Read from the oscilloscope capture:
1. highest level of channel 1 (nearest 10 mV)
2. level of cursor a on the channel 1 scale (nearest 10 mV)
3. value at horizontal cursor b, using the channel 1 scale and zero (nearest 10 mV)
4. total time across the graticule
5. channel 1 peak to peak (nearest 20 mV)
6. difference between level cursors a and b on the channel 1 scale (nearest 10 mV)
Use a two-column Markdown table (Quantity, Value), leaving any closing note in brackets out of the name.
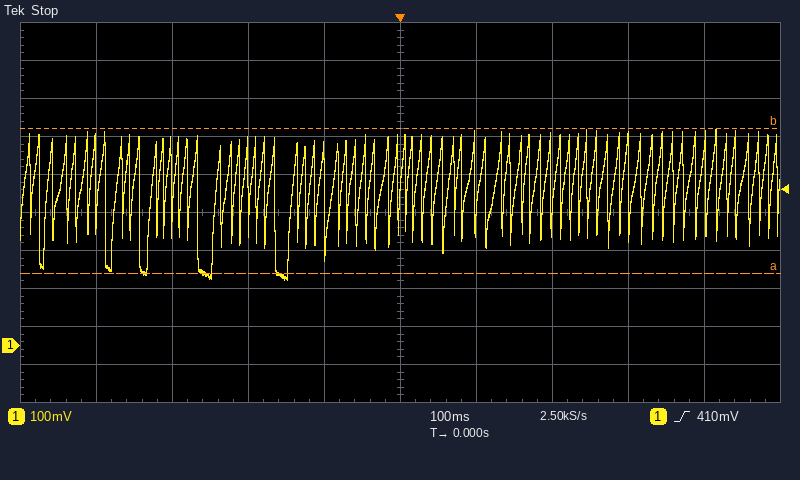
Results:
| Quantity | Value |
|---|---|
| highest level of channel 1 | 570 mV |
| level of cursor a on the channel 1 scale | 190 mV |
| value at horizontal cursor b, using the channel 1 scale and zero | 570 mV |
| total time across the graticule | 1 s |
| channel 1 peak to peak | 400 mV |
| difference between level cursors a and b on the channel 1 scale | 380 mV |
